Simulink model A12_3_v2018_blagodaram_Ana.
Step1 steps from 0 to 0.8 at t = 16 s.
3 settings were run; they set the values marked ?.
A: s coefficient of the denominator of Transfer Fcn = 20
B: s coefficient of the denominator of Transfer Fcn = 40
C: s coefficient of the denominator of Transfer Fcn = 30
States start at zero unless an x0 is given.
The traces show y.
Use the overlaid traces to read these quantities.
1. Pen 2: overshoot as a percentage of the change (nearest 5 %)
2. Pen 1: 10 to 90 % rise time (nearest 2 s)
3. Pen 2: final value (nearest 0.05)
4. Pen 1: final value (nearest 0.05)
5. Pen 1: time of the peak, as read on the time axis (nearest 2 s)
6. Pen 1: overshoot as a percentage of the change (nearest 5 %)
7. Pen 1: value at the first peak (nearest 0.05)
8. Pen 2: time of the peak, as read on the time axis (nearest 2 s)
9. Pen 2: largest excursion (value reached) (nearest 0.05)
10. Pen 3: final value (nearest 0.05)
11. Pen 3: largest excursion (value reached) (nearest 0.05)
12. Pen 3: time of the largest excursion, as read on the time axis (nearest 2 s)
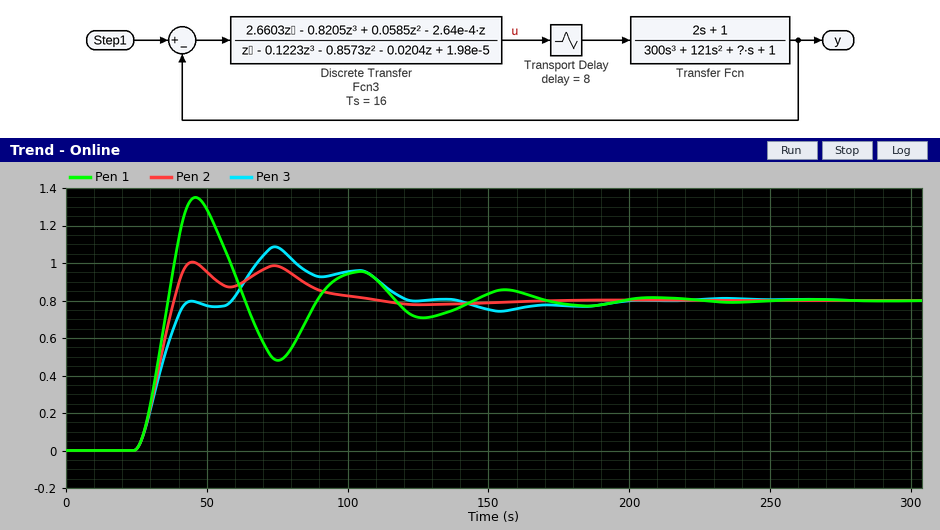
25 %
8 s
0.80
0.80
46 s
70 %
1.35
44 s
1.00
0.80
1.10
74 s
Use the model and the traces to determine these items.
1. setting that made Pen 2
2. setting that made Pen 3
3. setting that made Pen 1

C
B
A
